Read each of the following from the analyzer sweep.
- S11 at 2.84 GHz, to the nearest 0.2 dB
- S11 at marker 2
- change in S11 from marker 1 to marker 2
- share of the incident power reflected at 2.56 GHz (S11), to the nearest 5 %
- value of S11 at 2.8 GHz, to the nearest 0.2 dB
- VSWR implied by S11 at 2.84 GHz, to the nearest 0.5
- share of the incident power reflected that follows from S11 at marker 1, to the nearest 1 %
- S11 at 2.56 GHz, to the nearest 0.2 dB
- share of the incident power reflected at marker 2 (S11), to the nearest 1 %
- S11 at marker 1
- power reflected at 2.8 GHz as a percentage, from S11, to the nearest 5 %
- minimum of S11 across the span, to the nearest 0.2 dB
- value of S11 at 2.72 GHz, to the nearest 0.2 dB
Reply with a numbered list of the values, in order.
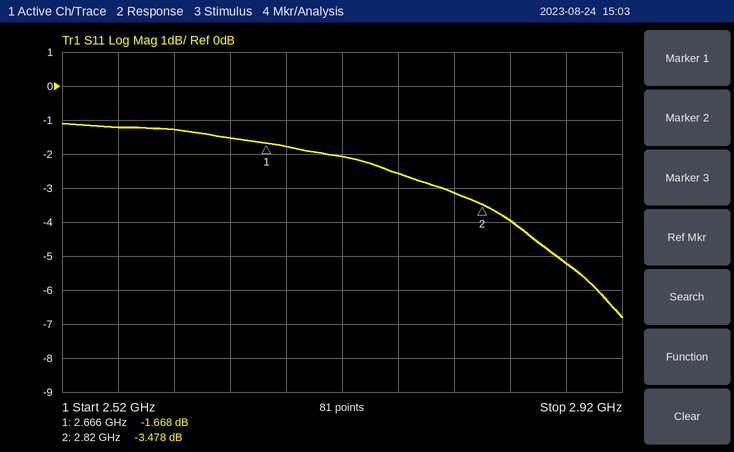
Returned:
1. -4.0 dB
2. -3.478 dB
3. -1.810 dB
4. 75 %
5. -3.2 dB
6. 4.5
7. 68 %
8. -1.2 dB
9. 45 %
10. -1.668 dB
11. 50 %
12. -6.8 dB
13. -2.0 dB
